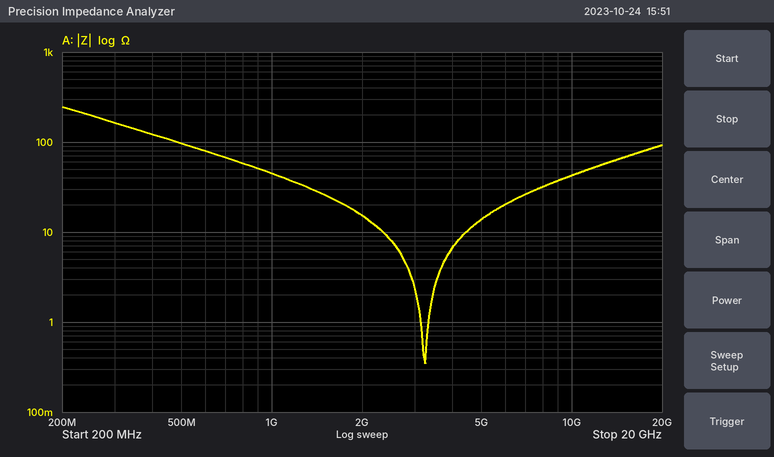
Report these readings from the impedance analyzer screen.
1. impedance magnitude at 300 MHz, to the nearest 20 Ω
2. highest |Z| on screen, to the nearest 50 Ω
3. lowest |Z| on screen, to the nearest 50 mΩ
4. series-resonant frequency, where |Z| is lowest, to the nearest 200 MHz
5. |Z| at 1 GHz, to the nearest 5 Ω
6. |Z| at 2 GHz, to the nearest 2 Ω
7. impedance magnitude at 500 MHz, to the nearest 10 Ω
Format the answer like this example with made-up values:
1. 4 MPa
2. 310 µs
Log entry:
1. 160 Ω
2. 250 Ω
3. 350 mΩ
4. 3.2 GHz
5. 45 Ω
6. 16 Ω
7. 100 Ω
